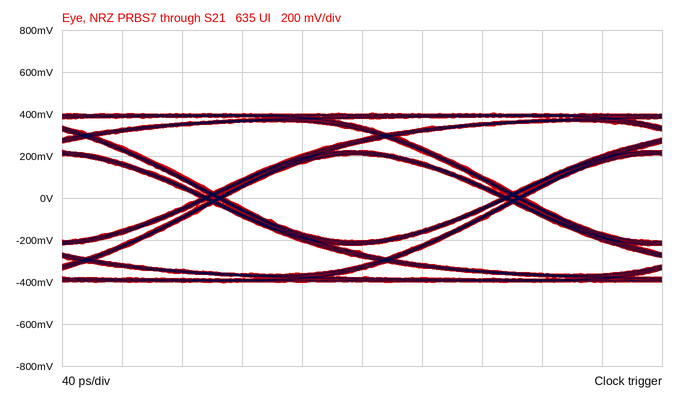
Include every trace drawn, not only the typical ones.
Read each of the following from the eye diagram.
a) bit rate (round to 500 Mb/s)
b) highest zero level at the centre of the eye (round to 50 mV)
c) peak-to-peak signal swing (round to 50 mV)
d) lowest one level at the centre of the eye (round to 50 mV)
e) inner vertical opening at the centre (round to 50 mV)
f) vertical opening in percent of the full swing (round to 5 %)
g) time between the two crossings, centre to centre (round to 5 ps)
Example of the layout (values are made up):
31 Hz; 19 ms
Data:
5.0 Gb/s; -200 mV; 800 mV; 200 mV; 400 mV; 50 %; 200 ps
